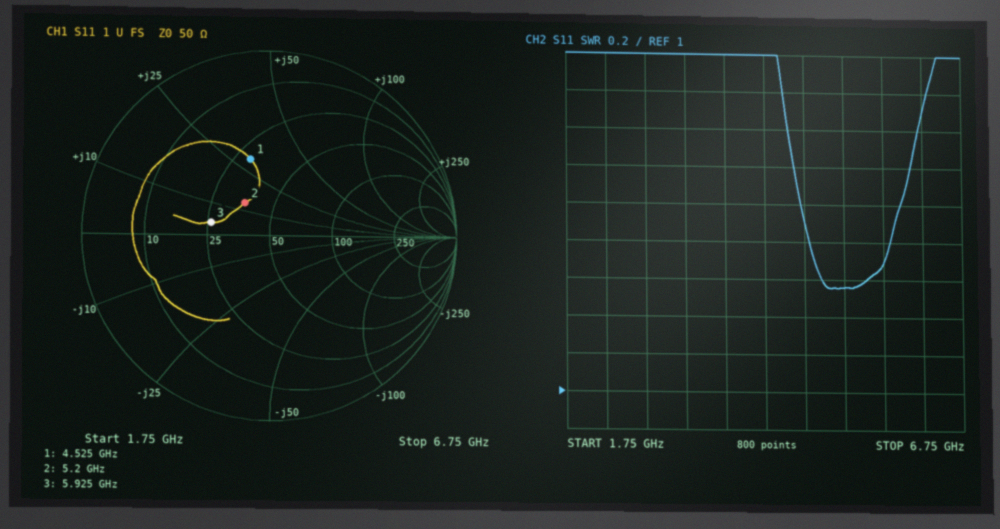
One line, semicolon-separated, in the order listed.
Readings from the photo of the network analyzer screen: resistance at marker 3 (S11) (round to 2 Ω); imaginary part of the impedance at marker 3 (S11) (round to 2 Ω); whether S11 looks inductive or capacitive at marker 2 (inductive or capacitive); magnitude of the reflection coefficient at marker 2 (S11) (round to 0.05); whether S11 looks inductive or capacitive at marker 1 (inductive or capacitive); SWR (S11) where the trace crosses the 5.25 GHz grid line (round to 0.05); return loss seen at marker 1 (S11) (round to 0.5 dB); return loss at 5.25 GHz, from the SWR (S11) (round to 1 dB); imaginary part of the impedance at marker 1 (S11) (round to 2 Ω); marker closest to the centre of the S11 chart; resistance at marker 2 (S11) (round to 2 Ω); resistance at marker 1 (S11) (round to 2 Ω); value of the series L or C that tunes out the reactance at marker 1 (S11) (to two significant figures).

26 Ω; +4 Ω; inductive; 0.20; inductive; 1.55; 7.5 dB; 13 dB; +30 Ω; marker 2; 36 Ω; 30 Ω; 1.2 pF
